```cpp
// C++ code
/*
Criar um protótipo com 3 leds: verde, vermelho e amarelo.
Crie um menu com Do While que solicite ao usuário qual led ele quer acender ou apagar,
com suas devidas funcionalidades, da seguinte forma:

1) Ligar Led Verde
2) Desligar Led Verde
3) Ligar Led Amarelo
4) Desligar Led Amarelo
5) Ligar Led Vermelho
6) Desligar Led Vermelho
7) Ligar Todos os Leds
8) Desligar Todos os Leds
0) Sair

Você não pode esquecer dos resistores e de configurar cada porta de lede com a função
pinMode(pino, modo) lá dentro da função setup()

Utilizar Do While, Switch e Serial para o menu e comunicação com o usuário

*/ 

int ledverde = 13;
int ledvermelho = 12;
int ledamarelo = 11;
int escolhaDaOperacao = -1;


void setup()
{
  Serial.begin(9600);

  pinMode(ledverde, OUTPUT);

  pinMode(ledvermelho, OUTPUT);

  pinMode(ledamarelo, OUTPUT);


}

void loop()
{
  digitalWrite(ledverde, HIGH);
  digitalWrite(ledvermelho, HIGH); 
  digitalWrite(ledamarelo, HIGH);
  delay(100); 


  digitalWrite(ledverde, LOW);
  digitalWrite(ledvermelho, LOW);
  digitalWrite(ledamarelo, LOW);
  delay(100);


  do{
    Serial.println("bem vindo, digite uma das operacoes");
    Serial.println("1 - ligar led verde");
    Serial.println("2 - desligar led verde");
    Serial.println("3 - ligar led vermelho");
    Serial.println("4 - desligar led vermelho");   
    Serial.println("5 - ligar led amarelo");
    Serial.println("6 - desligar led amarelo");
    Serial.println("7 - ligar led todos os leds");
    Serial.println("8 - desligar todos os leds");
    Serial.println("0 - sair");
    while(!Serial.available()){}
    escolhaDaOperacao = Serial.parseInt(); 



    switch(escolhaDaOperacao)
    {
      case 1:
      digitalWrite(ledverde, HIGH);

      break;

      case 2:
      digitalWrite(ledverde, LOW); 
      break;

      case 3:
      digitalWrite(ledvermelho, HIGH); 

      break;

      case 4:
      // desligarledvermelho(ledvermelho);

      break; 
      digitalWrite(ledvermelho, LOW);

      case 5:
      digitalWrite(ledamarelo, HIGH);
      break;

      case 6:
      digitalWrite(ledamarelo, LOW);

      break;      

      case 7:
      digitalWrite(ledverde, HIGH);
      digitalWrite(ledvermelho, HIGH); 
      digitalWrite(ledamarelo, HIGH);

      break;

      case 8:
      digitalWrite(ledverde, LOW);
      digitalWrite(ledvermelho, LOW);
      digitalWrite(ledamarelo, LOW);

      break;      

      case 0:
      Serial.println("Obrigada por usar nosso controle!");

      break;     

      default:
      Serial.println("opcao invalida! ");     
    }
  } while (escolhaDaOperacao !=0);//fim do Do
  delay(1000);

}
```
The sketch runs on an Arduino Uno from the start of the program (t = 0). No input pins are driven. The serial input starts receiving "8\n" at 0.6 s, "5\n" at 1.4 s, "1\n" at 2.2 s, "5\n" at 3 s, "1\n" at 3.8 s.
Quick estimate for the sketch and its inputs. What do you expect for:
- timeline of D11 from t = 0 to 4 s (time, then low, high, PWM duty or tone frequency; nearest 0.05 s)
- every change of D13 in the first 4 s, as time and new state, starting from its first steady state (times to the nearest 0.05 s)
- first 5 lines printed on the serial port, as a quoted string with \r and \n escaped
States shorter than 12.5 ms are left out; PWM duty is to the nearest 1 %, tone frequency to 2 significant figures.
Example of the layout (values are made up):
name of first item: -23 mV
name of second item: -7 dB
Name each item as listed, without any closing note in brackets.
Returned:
timeline of D11 from t = 0 to 4 s: 0 s high; 0.1 s low; 1.4 s high
every change of D13 in the first 4 s, as time and new state, starting from its first steady state: 0 s high; 0.1 s low; 2.2 s high
first 5 lines printed on the serial port, as a quoted string with \r and \n escaped: "bem vindo, digite uma das operacoes\r\n1 - ligar led verde\r\n2 - desligar led verde\r\n3 - ligar led vermelho\r\n4 - desligar led vermelho\r\n"
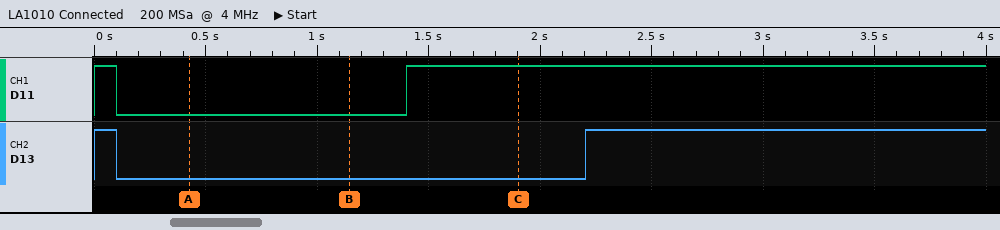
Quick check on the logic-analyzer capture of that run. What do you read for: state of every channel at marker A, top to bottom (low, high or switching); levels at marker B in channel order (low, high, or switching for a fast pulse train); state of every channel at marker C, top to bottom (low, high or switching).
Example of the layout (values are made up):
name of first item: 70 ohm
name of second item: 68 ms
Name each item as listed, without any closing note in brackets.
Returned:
state of every channel at marker A, top to bottom: D11 low, D13 low
levels at marker B in channel order: D11 low, D13 low
state of every channel at marker C, top to bottom: D11 high, D13 low
